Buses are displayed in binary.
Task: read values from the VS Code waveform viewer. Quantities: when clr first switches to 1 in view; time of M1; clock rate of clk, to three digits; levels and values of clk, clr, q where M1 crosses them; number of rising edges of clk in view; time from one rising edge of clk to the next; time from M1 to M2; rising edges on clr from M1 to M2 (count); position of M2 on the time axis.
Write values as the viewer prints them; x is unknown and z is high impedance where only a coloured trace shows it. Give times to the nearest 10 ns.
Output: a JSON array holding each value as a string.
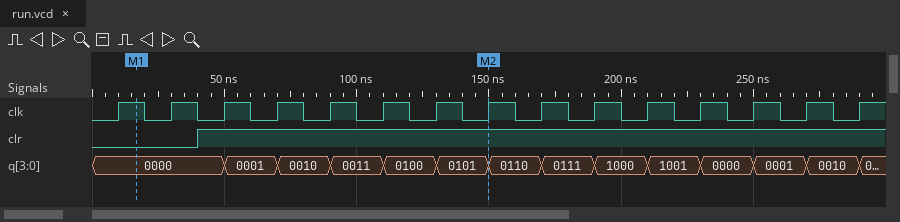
["40 ns", "20 ns", "50.0 MHz", "clk=1, clr=0, q=0000", "15", "20 ns", "130 ns", "1", "150 ns"]
